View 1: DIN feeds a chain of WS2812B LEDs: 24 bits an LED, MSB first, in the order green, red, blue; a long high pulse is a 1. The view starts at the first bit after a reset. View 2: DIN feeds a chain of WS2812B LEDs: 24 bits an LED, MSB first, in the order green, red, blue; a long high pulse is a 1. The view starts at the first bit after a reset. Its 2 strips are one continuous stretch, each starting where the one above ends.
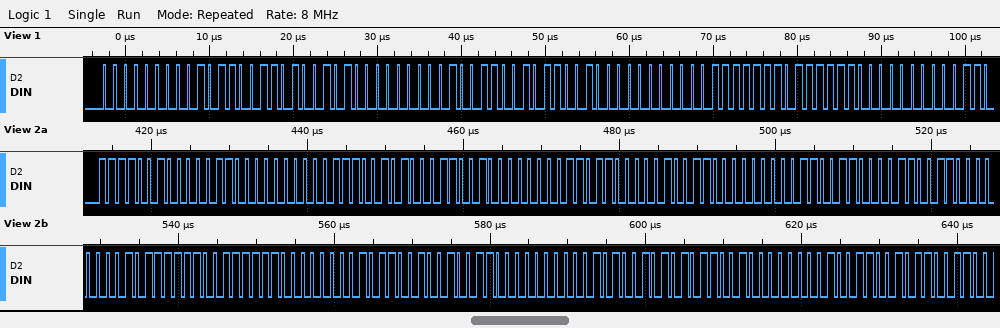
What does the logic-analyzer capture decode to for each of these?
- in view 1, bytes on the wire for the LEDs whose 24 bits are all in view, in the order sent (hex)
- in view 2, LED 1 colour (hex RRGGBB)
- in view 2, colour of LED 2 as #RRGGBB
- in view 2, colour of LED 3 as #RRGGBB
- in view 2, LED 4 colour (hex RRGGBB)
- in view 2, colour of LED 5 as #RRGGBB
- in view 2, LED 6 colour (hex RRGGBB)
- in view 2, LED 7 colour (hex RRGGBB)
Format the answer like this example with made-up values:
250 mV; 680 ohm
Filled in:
00 59 A5 00 4C B2 00 3F BF; #0CF200; #19E500; #26D800; #33CC00; #3FBF00; #4CB200; #59A500
